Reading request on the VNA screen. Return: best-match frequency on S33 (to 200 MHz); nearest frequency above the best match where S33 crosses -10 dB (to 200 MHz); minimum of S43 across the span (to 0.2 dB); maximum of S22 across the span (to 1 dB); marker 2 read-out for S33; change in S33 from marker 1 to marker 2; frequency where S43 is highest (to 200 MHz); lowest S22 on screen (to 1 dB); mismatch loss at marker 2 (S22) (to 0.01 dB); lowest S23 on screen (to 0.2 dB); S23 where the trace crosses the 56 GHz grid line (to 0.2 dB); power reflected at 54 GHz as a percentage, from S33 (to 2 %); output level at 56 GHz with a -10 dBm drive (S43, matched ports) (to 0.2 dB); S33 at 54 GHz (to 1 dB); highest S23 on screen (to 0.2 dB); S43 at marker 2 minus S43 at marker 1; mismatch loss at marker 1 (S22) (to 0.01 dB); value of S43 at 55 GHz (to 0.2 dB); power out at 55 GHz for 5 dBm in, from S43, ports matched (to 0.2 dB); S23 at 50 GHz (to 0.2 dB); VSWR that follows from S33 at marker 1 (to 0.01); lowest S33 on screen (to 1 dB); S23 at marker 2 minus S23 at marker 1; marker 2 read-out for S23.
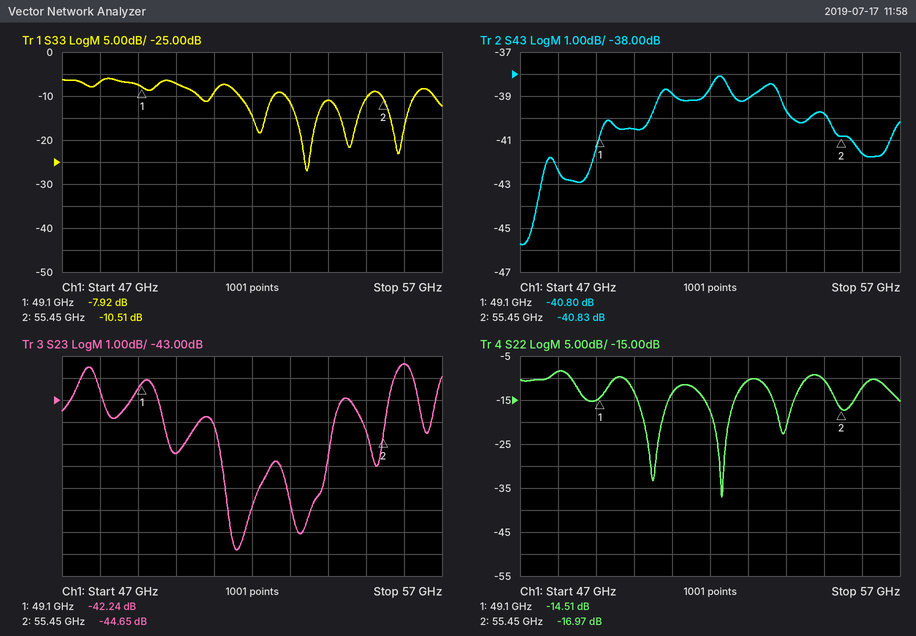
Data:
53.4 GHz
55.0 GHz
-45.8 dB
-8 dB
-10.51 dB
-2.59 dB
52.2 GHz
-37 dB
0.09 dB
-49.8 dB
-41.4 dB
8 %
-51.6 dBm
-11 dB
-41.4 dB
-0.03 dB
0.16 dB
-39.8 dB
-34.8 dBm
-45.4 dB
2.34
-27 dB
-2.41 dB
-44.65 dB
